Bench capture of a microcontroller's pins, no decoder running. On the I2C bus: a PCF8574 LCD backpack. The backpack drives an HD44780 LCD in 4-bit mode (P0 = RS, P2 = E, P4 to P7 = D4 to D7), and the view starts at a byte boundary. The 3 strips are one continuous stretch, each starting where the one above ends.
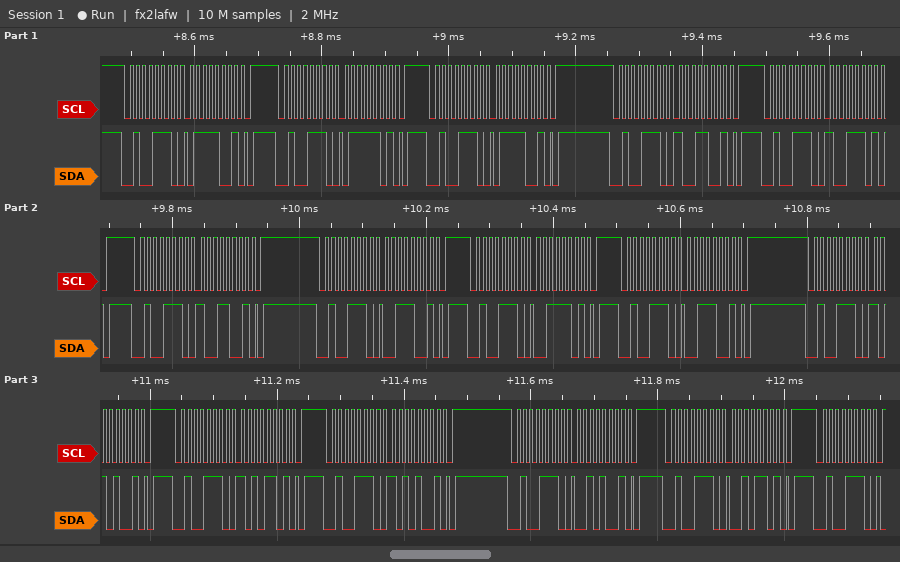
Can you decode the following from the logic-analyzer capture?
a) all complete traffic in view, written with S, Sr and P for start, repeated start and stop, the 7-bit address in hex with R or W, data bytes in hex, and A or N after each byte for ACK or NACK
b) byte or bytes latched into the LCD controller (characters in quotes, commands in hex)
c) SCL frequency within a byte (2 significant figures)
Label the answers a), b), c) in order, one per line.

a) S 27W A 79 A P S 27W A 7D A P S 27W A 79 A P S 27W A 99 A P S 27W A 9D A P S 27W A 99 A P S 27W A 39 A P S 27W A 3D A P S 27W A 39 A P S 27W A A9 A P S 27W A AD A P S 27W A A9 A P S 27W A 29 A P S 27W A 2D A P S 27W A
b) 'y' ':'
c) 100 kHz
